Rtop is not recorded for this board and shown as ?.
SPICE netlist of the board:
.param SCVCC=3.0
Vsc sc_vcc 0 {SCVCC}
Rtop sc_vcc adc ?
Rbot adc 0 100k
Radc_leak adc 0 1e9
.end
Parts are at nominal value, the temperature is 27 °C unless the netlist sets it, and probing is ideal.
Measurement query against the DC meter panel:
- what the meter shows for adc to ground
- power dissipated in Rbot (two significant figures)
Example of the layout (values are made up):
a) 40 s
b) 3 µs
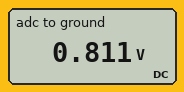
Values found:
a) 0.811 V
b) 6.6 µW
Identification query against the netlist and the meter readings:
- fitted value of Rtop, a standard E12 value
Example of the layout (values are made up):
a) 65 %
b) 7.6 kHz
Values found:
a) 270 kΩ
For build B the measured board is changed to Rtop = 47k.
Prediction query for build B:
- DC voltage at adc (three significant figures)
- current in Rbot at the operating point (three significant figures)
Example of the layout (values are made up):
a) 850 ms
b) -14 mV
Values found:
a) 2.04 V
b) 20.4 µA
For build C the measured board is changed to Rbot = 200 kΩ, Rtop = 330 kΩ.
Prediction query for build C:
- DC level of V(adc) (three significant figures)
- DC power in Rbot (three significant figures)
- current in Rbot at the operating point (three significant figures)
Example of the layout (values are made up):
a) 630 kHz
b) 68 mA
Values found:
a) 1.13 V
b) 6.41 µW
c) 5.66 µA
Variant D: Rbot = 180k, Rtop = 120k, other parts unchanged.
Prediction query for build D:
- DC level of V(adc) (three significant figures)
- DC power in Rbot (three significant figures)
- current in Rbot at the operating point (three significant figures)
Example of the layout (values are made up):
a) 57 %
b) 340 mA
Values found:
a) 1.80 V
b) 18.0 µW
c) 10.0 µA
